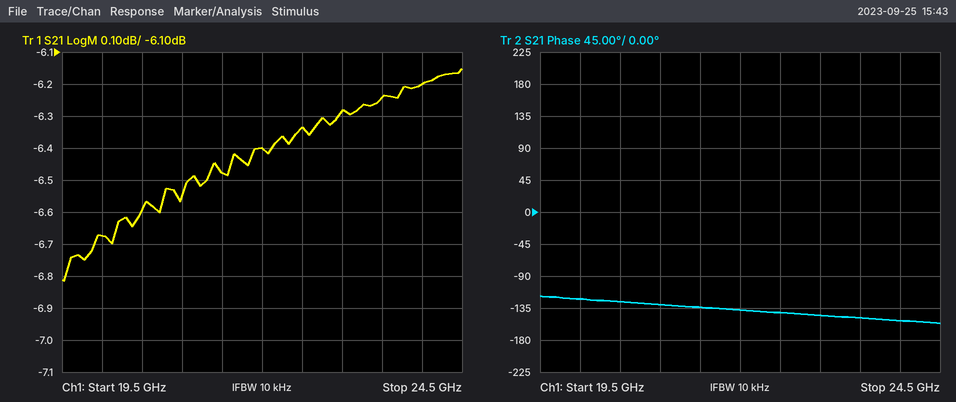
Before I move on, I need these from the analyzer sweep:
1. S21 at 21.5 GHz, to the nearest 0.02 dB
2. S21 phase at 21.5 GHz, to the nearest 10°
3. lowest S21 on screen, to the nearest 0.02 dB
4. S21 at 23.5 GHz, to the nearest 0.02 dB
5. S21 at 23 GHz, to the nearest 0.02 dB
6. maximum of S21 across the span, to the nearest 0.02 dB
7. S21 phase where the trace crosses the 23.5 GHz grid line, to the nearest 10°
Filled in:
-6.48 dB
-130°
-6.82 dB
-6.24 dB
-6.28 dB
-6.16 dB
-150°
